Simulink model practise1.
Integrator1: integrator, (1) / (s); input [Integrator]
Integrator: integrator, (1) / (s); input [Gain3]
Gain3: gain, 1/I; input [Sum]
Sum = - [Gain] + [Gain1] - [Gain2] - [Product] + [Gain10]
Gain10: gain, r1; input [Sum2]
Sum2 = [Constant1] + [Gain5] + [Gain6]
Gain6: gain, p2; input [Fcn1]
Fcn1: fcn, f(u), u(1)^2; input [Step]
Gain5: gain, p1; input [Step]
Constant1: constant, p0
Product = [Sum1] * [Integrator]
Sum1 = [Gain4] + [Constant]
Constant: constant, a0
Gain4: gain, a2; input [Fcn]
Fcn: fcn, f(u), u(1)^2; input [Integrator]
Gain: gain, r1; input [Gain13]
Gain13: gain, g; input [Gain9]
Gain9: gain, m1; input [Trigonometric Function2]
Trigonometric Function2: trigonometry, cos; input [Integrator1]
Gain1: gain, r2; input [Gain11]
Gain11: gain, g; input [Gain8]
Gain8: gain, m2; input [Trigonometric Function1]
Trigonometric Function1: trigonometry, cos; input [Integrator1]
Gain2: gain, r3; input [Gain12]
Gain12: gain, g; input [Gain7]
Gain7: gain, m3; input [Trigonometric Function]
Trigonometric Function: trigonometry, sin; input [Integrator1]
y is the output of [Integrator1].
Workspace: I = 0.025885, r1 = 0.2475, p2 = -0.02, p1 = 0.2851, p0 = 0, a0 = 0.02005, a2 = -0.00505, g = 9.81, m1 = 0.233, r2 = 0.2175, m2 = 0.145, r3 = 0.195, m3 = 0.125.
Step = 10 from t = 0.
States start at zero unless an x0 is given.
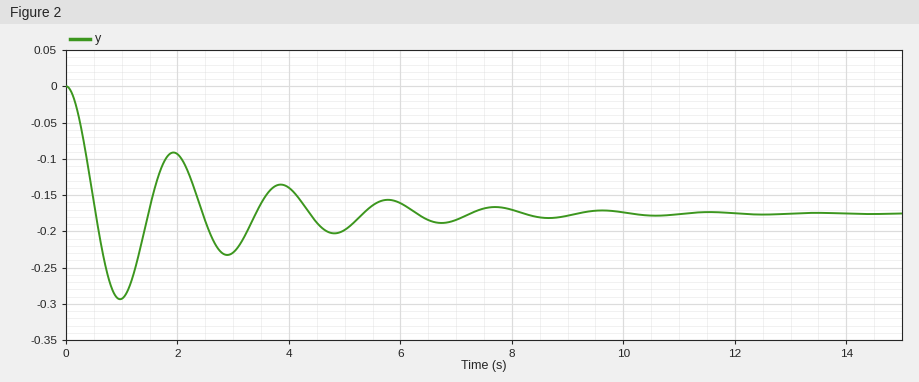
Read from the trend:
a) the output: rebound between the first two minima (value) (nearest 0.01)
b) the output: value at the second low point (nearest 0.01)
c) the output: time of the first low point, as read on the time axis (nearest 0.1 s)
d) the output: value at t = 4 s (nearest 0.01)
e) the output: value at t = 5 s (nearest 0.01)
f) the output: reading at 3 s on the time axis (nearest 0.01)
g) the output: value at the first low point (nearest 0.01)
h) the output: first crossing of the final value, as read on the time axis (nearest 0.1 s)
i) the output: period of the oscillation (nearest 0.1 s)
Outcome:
-0.09
-0.23
1.0 s
-0.14
-0.20
-0.23
-0.29
0.5 s
1.9 s
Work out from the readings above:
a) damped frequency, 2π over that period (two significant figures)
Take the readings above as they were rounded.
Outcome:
3.3 rad/s
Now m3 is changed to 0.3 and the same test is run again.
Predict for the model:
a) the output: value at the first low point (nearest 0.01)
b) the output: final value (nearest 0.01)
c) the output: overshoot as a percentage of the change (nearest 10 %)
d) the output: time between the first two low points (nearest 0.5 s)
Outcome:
-0.14
-0.08
80 %
1.5 s
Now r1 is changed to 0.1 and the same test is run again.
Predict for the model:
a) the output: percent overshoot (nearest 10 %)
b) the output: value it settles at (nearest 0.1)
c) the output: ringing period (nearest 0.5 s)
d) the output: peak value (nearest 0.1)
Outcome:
100 %
0.7
2.0 s
1.3
